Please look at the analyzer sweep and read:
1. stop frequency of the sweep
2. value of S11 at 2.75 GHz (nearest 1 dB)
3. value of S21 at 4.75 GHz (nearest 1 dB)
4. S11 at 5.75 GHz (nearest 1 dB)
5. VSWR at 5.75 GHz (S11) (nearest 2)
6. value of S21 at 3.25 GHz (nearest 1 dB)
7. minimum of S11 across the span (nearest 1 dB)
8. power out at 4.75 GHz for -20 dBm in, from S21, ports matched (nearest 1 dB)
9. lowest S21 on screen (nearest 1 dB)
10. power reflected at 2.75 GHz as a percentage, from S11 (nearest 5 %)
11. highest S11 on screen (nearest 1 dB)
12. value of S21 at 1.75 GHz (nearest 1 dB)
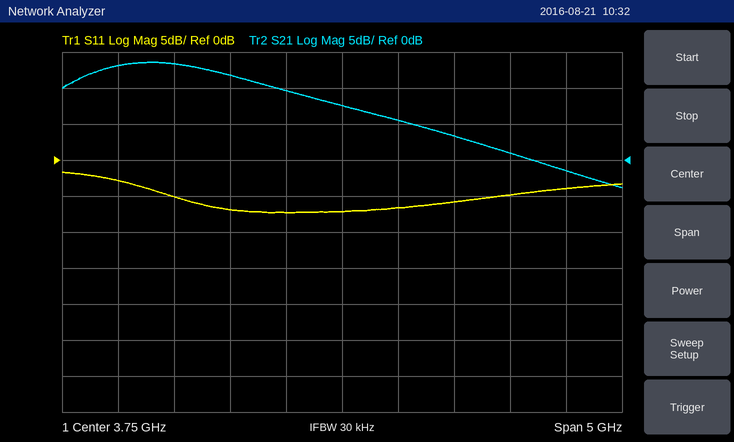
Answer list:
6.25 GHz
-7 dB
3 dB
-4 dB
4
10 dB
-7 dB
-17 dBm
-4 dB
20 %
-2 dB
13 dB
